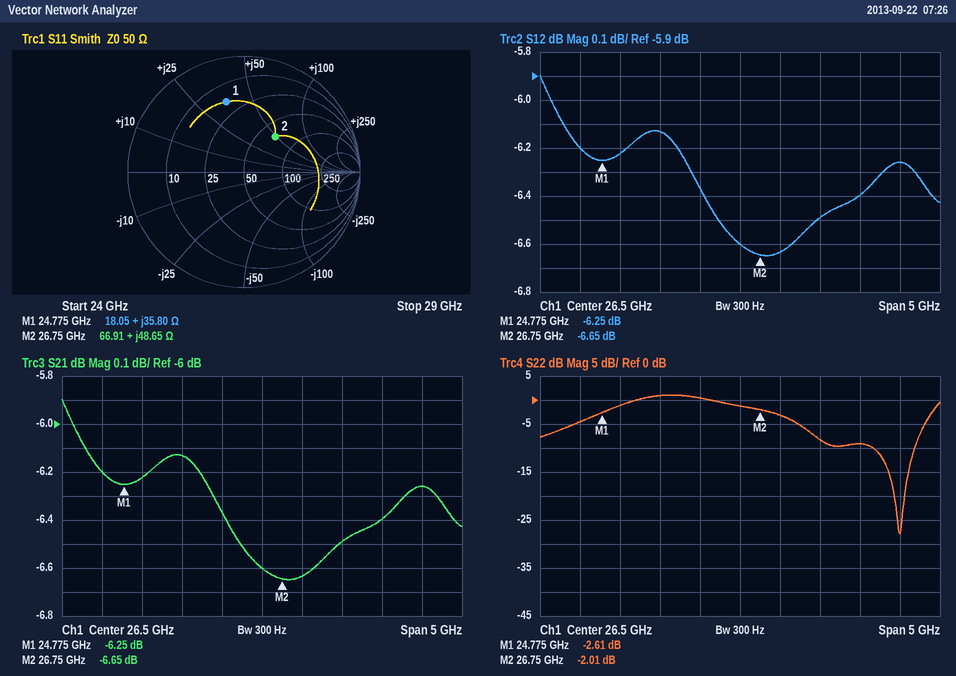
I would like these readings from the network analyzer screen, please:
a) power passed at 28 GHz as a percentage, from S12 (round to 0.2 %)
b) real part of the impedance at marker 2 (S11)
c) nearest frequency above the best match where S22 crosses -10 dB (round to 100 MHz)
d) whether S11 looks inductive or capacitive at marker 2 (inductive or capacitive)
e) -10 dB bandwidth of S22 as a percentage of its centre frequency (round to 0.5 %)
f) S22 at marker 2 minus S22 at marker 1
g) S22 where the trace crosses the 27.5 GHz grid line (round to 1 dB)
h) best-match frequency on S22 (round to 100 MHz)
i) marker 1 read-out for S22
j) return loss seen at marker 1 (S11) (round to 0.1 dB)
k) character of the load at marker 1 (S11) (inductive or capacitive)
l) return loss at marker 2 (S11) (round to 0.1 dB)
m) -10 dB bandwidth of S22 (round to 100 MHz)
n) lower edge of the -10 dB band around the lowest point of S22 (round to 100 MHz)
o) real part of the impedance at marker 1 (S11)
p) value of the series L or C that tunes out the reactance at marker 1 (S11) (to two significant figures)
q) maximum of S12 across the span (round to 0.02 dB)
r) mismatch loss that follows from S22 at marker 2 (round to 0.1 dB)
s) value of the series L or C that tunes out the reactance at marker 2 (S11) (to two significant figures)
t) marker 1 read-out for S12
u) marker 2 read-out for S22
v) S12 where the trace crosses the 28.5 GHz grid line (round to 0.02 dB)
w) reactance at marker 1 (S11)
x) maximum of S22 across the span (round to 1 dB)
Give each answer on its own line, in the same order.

23.0 %
66.91 Ω
28.7 GHz
inductive
2.0 %
0.60 dB
-8 dB
28.5 GHz
-2.61 dB
4.1 dB
inductive
7.8 dB
500 MHz
28.2 GHz
18.05 Ω
180 fF
-5.90 dB
4.3 dB
120 fF
-6.25 dB
-2.01 dB
-6.26 dB
+35.80 Ω
1 dB
